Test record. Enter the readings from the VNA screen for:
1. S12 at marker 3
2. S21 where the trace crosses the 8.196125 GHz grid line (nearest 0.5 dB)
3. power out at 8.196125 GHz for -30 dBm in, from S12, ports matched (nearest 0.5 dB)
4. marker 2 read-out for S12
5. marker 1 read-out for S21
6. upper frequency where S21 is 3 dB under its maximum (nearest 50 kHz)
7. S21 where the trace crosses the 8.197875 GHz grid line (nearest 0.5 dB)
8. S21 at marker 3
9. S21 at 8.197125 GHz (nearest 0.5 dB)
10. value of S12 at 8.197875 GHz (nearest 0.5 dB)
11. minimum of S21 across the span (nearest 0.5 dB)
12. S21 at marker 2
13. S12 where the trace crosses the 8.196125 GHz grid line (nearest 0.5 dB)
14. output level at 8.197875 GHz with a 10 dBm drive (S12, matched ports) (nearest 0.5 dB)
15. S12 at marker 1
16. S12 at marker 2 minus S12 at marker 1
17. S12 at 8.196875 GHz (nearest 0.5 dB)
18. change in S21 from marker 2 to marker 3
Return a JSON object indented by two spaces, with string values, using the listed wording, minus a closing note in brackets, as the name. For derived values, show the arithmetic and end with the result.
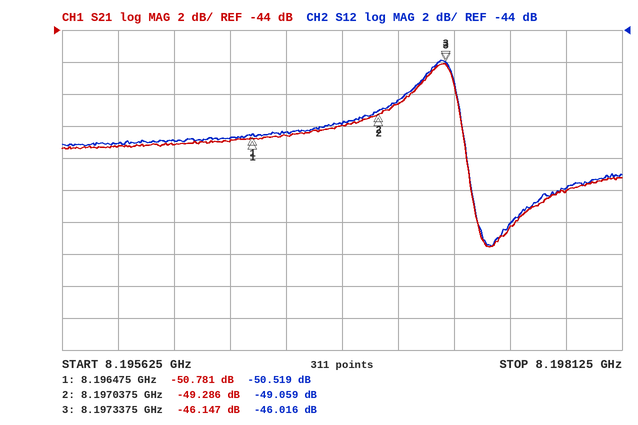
{
  "S12 at marker 3": "-46.016 dB",
  "S21 where the trace crosses the 8.196125 GHz grid line": "-51.0 dB",
  "power out at 8.196125 GHz for -30 dBm in, from S12, ports matched": "-30 dBm + (-51.0 dB) = -81.0 dBm",
  "marker 2 read-out for S12": "-49.059 dB",
  "marker 1 read-out for S21": "-50.781 dB",
  "upper frequency where S21 is 3 dB under its maximum": "8.19740 GHz",
  "S21 where the trace crosses the 8.197875 GHz grid line": "-54.0 dB",
  "S21 at marker 3": "-46.147 dB",
  "S21 at 8.197125 GHz": "-48.5 dB",
  "value of S12 at 8.197875 GHz": "-54.0 dB",
  "minimum of S21 across the span": "-57.5 dB",
  "S21 at marker 2": "-49.286 dB",
  "S12 where the trace crosses the 8.196125 GHz grid line": "-51.0 dB",
  "output level at 8.197875 GHz with a 10 dBm drive (S12, matched ports)": "10 dBm + (-54.0 dB) = -44.0 dBm",
  "S12 at marker 1": "-50.519 dB",
  "S12 at marker 2 minus S12 at marker 1": "-49.059 − (-50.519) = 1.460 dB",
  "S12 at 8.196875 GHz": "-50.0 dB",
  "change in S21 from marker 2 to marker 3": "-46.147 − (-49.286) = 3.139 dB"
}
